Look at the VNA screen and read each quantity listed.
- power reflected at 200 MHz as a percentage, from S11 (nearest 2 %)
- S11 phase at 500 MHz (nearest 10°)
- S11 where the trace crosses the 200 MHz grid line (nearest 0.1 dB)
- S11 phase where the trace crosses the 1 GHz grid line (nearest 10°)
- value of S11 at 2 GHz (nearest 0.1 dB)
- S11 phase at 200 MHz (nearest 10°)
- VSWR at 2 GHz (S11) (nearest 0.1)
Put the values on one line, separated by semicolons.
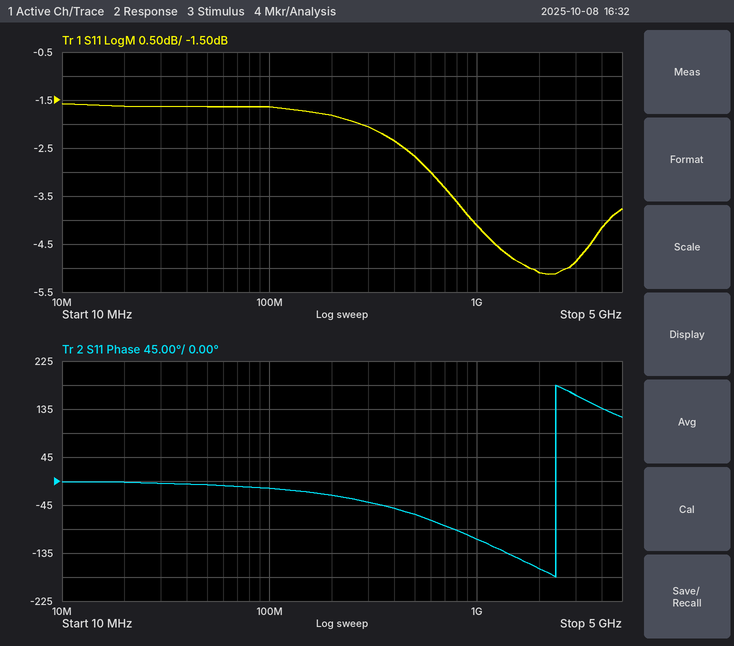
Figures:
66 %; -60°; -1.8 dB; -110°; -5.1 dB; -30°; 3.5
